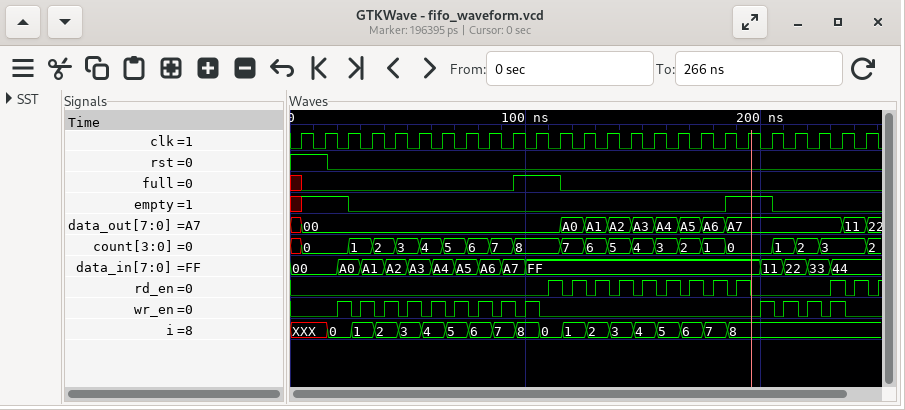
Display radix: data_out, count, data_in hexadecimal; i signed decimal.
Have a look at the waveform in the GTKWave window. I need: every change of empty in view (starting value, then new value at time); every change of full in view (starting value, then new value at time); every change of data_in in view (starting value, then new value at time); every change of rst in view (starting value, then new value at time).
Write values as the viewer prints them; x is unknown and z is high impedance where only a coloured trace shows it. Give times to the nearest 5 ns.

x, 1 at 5 ns, 0 at 25 ns, 1 at 185 ns, 0 at 205 ns
x, 0 at 5 ns, 1 at 95 ns, 0 at 115 ns
00, A0 at 20 ns, A1 at 30 ns, A2 at 40 ns, A3 at 50 ns, A4 at 60 ns, A5 at 70 ns, A6 at 80 ns, A7 at 90 ns, FF at 100 ns, 11 at 200 ns, 22 at 210 ns, 33 at 220 ns, 44 at 230 ns
1, 0 at 15 ns
